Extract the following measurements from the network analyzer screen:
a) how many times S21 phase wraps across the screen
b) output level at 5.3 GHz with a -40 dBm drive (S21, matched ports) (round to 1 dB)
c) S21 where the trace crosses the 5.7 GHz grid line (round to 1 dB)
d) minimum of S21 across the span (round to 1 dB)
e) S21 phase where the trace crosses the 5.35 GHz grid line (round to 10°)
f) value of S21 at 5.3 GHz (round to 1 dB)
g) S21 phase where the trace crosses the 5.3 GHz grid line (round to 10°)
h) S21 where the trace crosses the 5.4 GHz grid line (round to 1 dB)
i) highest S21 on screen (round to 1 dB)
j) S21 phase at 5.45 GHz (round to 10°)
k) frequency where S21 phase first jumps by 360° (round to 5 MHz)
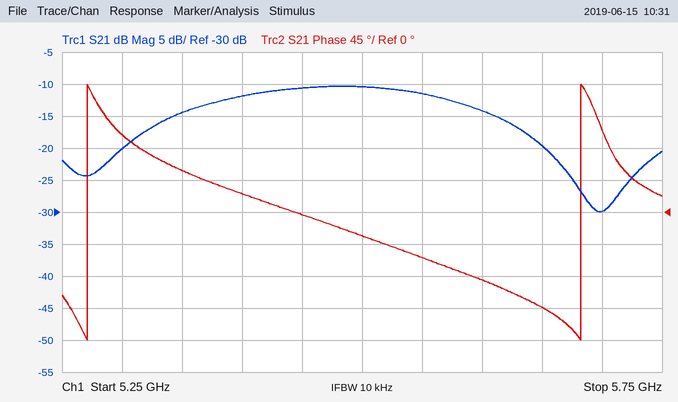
2
-60 dBm
-30 dB
-30 dB
60°
-20 dB
110°
-12 dB
-10 dB
0°
5.270 GHz
